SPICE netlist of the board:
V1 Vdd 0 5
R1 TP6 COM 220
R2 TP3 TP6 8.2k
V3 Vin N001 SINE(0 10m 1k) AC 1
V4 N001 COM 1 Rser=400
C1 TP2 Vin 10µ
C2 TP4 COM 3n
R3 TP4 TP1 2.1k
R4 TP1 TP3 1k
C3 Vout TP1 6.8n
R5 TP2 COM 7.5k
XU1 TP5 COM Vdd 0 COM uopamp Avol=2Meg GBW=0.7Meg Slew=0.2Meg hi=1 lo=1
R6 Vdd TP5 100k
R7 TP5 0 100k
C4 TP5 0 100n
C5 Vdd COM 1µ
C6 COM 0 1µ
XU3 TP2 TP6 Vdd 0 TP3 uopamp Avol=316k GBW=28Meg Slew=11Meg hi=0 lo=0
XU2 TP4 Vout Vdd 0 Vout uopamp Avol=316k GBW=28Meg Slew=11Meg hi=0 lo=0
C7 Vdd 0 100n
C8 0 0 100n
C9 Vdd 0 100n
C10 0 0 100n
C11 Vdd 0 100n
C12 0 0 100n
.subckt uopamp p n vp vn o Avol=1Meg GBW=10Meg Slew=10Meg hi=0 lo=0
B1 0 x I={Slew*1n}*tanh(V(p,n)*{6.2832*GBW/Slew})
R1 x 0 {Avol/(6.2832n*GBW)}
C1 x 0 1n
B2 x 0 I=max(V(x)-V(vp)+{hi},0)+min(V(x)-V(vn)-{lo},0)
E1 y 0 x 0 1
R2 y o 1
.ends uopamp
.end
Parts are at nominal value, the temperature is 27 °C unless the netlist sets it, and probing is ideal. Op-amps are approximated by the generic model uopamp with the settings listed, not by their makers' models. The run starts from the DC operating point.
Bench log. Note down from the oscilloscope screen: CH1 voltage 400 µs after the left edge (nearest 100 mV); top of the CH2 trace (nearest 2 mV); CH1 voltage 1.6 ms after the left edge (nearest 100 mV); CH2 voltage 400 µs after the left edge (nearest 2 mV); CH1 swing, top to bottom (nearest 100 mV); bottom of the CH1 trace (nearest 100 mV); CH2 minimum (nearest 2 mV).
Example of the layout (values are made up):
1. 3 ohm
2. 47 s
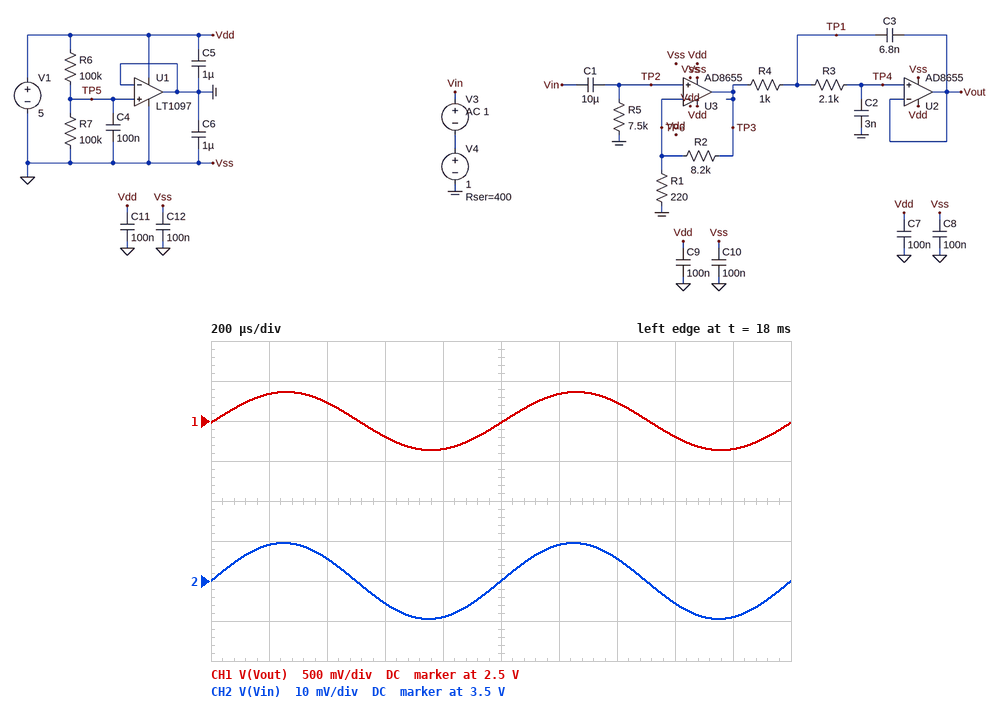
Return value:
1. 2.7 V
2. 3.510 V
3. 2.3 V
4. 3.506 V
5. 700 mV
6. 2.1 V
7. 3.490 V
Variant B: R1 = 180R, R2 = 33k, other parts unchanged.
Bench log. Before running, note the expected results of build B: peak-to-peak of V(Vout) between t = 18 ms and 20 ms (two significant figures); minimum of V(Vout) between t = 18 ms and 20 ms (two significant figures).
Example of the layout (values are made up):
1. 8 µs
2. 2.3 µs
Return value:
1. 3.5 V
2. 750 mV
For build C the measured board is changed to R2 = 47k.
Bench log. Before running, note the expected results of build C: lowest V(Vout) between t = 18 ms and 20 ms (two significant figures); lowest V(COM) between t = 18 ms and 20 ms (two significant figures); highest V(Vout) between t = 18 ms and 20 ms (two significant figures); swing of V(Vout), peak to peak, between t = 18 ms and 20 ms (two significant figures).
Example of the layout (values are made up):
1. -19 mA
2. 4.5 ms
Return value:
1. 460 mV
2. 2.5 V
3. 4.5 V
4. 4.1 V
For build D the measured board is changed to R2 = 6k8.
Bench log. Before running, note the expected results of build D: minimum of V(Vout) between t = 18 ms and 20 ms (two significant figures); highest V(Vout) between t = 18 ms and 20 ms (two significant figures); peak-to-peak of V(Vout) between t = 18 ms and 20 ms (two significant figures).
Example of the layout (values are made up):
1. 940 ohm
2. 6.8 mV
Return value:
1. 2.2 V
2. 2.8 V
3. 610 mV
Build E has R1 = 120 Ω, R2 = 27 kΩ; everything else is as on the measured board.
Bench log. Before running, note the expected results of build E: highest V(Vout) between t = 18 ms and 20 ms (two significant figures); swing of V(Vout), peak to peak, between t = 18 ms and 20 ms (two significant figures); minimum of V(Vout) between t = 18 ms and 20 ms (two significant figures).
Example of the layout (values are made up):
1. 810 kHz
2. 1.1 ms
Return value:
1. 4.6 V
2. 4.3 V
3. 350 mV
